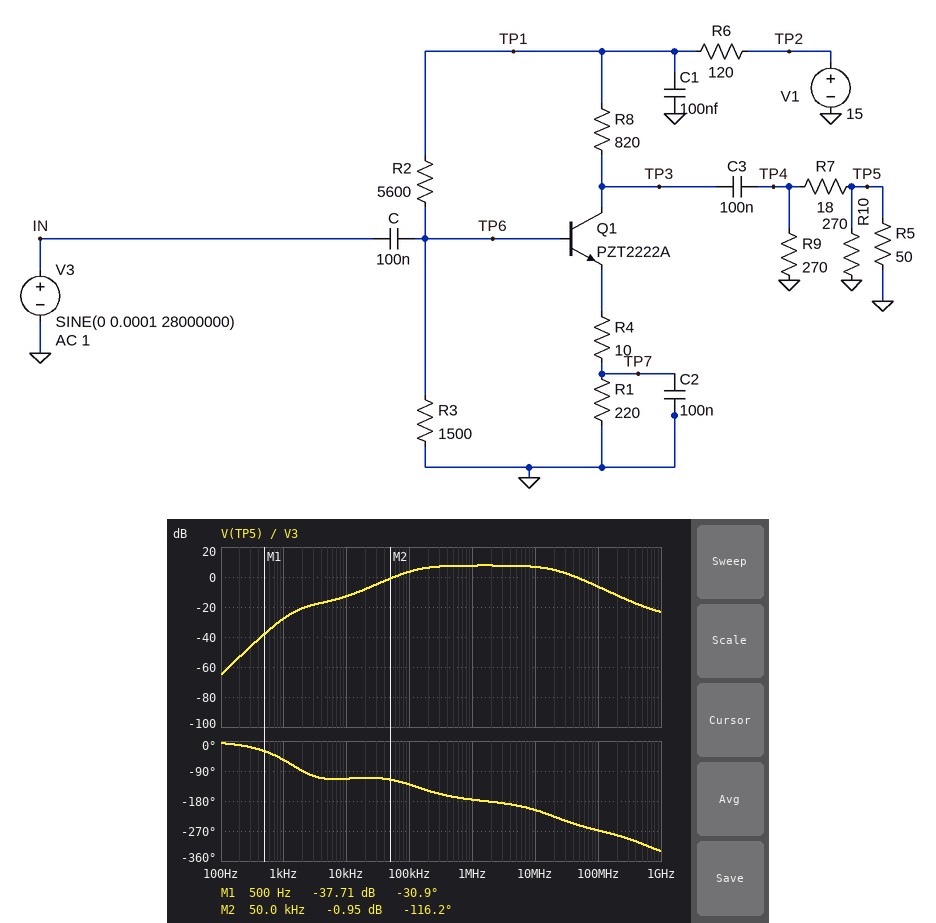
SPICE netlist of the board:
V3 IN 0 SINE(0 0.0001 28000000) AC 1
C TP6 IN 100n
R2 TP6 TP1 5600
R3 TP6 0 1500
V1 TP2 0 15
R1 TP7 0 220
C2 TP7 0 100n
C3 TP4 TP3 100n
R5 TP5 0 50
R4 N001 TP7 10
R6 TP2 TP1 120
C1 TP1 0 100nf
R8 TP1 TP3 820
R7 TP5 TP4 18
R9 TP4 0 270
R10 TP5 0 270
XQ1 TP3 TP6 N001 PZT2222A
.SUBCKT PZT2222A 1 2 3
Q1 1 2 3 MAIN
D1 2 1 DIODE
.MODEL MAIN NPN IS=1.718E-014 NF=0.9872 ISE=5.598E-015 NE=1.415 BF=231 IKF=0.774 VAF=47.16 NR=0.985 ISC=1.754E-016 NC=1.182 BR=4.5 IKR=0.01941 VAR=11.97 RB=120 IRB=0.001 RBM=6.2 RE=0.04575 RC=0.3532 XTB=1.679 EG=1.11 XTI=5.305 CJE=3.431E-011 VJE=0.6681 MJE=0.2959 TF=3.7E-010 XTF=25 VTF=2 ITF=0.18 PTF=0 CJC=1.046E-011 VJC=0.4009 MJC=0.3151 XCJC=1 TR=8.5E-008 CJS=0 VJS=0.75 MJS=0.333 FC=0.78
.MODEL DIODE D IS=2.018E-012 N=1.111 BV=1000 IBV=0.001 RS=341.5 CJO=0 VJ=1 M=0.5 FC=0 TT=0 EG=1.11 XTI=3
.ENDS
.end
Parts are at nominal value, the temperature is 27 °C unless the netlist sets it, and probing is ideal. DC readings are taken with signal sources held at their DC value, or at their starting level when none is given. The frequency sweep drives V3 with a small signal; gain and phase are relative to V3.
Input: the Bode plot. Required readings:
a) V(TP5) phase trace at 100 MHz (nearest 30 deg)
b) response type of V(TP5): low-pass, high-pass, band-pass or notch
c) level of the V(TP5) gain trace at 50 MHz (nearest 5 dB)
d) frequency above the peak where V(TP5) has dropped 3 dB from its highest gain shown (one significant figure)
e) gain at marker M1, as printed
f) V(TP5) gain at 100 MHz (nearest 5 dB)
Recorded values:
-270 deg
band-pass
0 dB
20 MHz
-37.71 dB
-5 dB
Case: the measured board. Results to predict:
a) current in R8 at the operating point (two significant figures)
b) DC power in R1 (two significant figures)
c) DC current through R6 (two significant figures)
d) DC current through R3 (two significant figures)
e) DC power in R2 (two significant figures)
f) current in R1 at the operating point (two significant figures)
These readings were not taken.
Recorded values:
9.3 mA
19 mW
11 mA
1.9 mA
21 mW
9.3 mA
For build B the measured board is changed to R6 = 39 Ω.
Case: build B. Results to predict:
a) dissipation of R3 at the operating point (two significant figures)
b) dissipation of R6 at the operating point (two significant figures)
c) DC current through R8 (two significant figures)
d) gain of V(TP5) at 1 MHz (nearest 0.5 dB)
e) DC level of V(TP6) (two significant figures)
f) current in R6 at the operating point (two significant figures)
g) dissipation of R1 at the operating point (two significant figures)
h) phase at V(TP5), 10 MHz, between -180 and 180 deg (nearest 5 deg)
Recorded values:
6.1 mW
5.7 mW
10 mA
8.0 dB
3.0 V
12 mA
22 mW
155 deg
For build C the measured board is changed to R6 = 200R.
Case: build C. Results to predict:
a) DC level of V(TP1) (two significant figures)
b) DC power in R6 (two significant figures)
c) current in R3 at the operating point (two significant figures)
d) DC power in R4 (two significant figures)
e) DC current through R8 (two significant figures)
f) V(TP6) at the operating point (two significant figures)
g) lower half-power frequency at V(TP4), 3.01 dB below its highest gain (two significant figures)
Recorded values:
13 V
22 mW
1.8 mA
750 µW
8.6 mA
2.7 V
120 kHz
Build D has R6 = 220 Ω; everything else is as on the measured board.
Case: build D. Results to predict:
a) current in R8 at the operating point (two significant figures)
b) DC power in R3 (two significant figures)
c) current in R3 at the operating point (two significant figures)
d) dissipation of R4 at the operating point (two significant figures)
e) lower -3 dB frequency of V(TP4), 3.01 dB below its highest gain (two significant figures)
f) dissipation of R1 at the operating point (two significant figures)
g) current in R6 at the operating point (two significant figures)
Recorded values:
8.5 mA
4.7 mW
1.8 mA
720 µW
120 kHz
16 mW
10 mA
